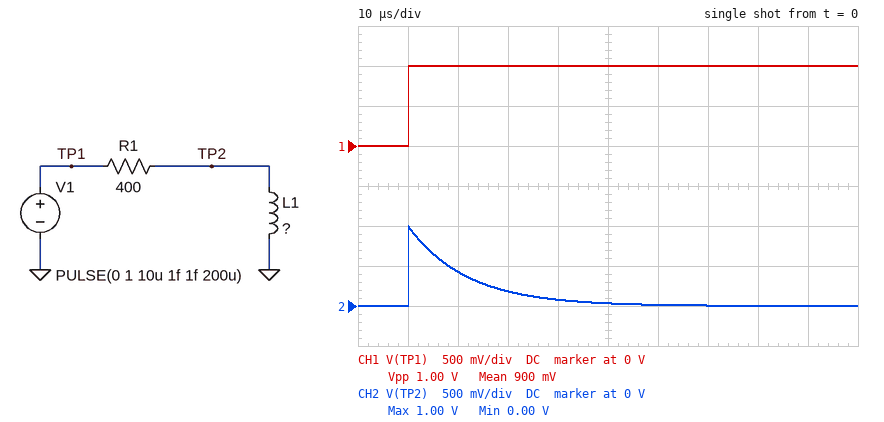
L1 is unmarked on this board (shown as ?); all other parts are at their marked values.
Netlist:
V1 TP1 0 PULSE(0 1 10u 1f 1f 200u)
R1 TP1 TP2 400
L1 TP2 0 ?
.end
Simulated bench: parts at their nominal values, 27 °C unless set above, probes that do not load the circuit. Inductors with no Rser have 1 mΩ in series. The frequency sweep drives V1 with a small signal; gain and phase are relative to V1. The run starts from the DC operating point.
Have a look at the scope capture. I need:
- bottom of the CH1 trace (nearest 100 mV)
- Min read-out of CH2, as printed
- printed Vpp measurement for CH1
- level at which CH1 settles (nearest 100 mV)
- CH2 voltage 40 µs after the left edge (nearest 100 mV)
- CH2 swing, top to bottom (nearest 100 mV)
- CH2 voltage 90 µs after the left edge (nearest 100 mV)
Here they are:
0 V
0.00 V
1.00 V
1.0 V
100 mV
1.0 V
0 V
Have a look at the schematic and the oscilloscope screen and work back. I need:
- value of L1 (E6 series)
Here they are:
4.7 mH
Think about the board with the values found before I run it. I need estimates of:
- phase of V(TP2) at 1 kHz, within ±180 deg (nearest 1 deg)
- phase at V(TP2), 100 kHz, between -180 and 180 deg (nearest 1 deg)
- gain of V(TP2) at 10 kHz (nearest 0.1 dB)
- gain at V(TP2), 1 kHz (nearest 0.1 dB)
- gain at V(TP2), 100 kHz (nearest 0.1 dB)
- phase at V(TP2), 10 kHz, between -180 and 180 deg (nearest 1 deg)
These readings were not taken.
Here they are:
86 deg
8 deg
-4.5 dB
-22.7 dB
-0.1 dB
54 deg
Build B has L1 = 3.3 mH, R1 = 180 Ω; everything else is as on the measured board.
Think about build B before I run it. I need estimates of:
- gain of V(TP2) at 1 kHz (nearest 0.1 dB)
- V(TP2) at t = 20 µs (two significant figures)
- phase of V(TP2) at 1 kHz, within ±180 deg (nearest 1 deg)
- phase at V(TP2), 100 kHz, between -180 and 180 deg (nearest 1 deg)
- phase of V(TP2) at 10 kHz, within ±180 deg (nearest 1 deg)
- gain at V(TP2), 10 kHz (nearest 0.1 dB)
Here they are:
-18.8 dB
580 mV
83 deg
5 deg
41 deg
-2.4 dB
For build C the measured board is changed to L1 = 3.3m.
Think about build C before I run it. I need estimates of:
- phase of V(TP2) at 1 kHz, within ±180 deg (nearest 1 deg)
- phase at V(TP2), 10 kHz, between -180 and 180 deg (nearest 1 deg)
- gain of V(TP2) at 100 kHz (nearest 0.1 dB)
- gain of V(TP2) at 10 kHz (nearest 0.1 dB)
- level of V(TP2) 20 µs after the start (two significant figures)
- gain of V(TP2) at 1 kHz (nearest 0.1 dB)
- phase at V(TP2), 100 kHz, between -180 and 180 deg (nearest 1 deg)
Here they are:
87 deg
63 deg
-0.2 dB
-6.7 dB
300 mV
-25.7 dB
11 deg
